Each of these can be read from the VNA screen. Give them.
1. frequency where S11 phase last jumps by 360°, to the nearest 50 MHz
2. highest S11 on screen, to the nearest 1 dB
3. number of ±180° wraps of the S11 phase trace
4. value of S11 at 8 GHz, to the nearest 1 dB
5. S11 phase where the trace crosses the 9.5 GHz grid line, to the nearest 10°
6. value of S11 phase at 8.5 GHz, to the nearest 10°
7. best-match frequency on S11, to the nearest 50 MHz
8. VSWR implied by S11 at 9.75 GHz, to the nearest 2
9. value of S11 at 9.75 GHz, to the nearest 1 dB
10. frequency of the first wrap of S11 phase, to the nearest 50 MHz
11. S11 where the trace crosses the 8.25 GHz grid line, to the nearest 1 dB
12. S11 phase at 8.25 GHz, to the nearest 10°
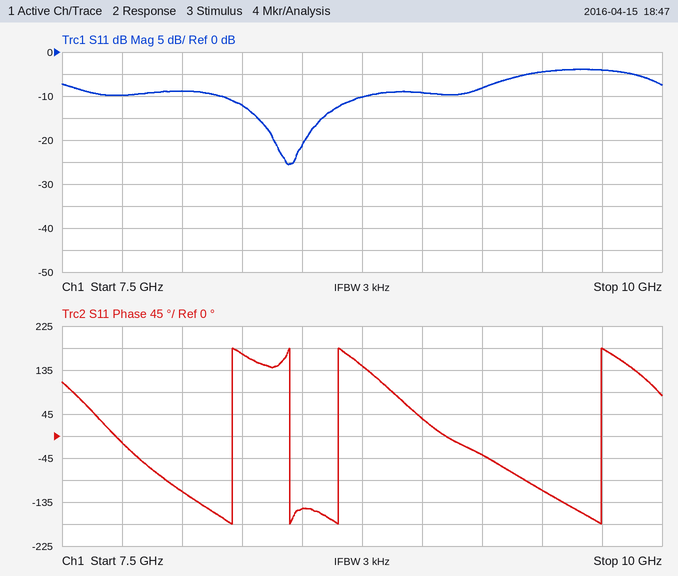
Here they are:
9.75 GHz
-4 dB
4
-9 dB
-110°
-150°
8.45 GHz
4
-4 dB
8.20 GHz
-12 dB
170°
